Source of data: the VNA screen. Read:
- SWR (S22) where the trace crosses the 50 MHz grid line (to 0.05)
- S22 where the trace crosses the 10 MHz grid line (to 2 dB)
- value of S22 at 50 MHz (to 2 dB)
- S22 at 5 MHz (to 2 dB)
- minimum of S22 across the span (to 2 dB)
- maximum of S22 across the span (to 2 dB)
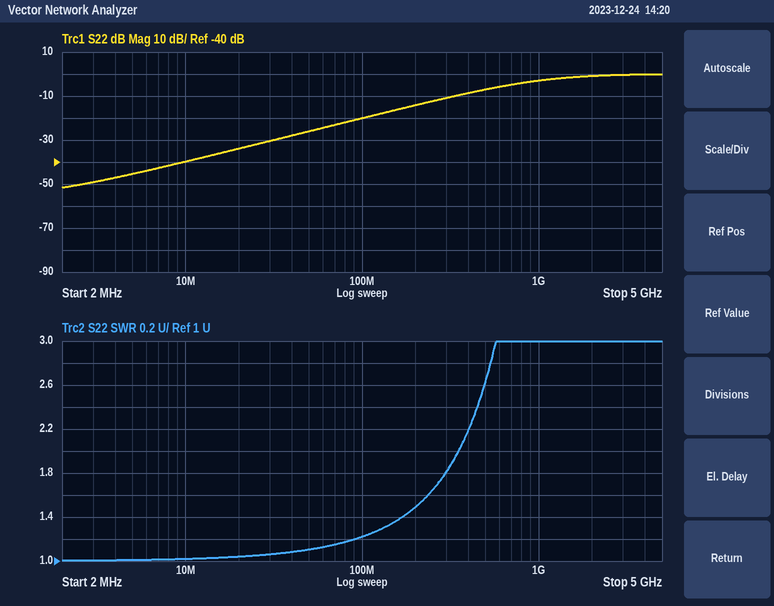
1.10
-40 dB
-26 dB
-46 dB
-52 dB
0 dB
